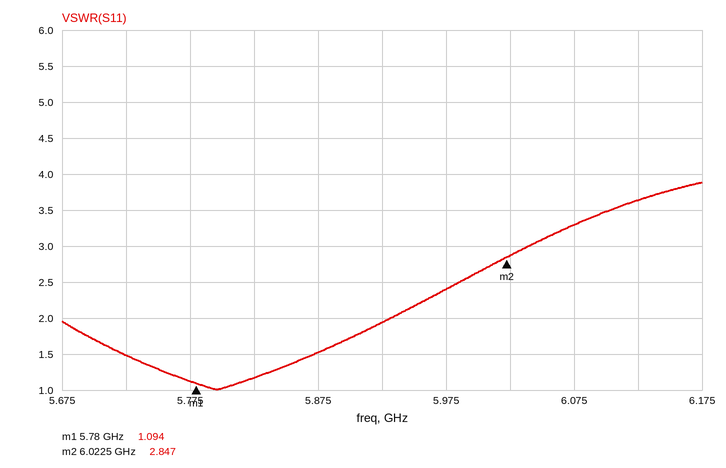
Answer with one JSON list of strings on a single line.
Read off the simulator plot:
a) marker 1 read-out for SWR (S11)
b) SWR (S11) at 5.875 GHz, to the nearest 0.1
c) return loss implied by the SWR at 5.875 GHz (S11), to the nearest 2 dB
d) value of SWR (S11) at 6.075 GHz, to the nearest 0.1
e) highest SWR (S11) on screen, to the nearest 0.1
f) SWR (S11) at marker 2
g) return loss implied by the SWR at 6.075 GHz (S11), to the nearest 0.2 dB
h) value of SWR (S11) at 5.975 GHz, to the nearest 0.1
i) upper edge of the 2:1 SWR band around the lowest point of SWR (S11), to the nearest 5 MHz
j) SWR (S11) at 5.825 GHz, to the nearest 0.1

["1.094", "1.5", "14 dB", "3.3", "3.9", "2.847", "5.4 dB", "2.4", "5.930 GHz", "1.2"]
